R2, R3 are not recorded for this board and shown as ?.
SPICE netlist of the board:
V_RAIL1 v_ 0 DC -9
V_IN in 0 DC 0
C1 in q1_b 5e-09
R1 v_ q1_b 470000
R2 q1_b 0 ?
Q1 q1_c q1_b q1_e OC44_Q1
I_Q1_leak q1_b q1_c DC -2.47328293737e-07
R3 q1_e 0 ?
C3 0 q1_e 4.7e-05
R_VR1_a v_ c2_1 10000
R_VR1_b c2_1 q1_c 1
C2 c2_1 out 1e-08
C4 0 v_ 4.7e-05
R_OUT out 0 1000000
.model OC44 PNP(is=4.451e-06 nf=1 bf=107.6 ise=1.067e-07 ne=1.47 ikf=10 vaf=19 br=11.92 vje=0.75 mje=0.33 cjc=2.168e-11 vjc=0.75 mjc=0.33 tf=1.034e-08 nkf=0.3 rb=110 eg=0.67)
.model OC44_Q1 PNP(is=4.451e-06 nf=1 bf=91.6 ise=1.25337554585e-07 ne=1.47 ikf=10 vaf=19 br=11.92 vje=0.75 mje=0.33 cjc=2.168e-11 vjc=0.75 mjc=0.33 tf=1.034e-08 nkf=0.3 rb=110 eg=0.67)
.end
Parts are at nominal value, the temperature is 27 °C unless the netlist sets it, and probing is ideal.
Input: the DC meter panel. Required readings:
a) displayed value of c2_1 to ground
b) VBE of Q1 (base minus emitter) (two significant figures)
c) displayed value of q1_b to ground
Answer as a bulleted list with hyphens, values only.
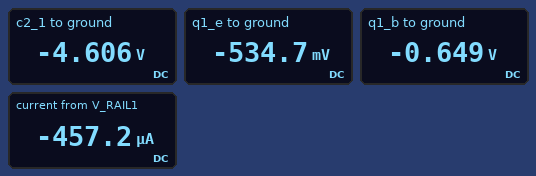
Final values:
- -4.606 V
- -110 mV
- -0.649 V
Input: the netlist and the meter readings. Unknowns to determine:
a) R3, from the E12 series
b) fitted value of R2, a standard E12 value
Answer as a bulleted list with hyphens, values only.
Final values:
- 1.2 kΩ
- 56 kΩ
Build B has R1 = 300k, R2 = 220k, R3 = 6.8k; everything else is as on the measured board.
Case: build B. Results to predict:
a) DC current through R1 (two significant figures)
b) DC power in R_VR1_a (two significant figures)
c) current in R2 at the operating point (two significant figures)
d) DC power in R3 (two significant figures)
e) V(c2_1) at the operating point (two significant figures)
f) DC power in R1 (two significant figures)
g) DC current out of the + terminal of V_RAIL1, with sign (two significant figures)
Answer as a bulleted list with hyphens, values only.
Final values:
- 20 µA
- 1.7 mW
- 14 µA
- 1.2 mW
- -4.8 V
- 120 µW
- -440 µA
